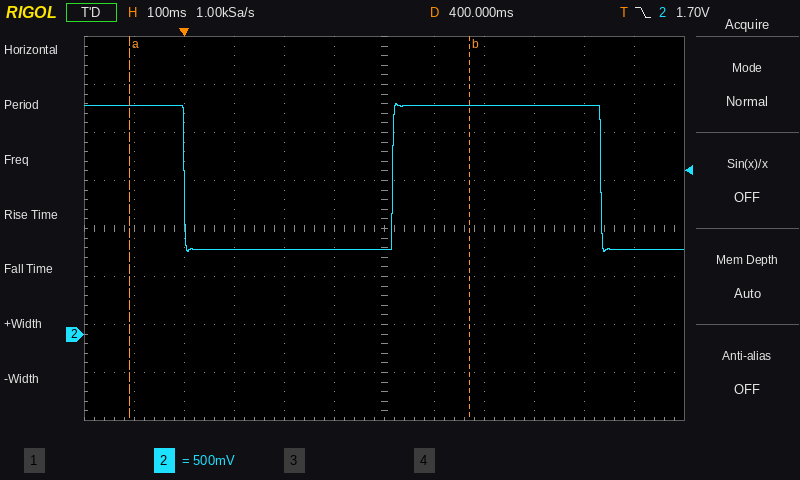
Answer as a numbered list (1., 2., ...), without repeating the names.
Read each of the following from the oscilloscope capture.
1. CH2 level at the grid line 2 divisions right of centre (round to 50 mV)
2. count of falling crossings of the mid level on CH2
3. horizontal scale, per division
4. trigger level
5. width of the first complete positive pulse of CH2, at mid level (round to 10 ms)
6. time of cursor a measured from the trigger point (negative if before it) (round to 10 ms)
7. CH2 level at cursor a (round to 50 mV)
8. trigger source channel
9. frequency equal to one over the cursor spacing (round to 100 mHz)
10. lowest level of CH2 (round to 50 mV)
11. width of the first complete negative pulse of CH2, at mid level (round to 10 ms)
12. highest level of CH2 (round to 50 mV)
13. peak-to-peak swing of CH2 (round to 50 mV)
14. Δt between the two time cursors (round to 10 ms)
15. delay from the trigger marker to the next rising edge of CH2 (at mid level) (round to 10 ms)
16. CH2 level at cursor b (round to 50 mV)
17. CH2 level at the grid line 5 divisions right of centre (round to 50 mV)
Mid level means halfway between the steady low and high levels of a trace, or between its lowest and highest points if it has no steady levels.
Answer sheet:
1. 2.40 V
2. 2
3. 100 ms
4. 1.70 V
5. 420 ms
6. -110 ms
7. 2.40 V
8. CH2
9. 1.5 Hz
10. 850 mV
11. 420 ms
12. 2.40 V
13. 1.55 V
14. 680 ms
15. 420 ms
16. 2.40 V
17. 900 mV
